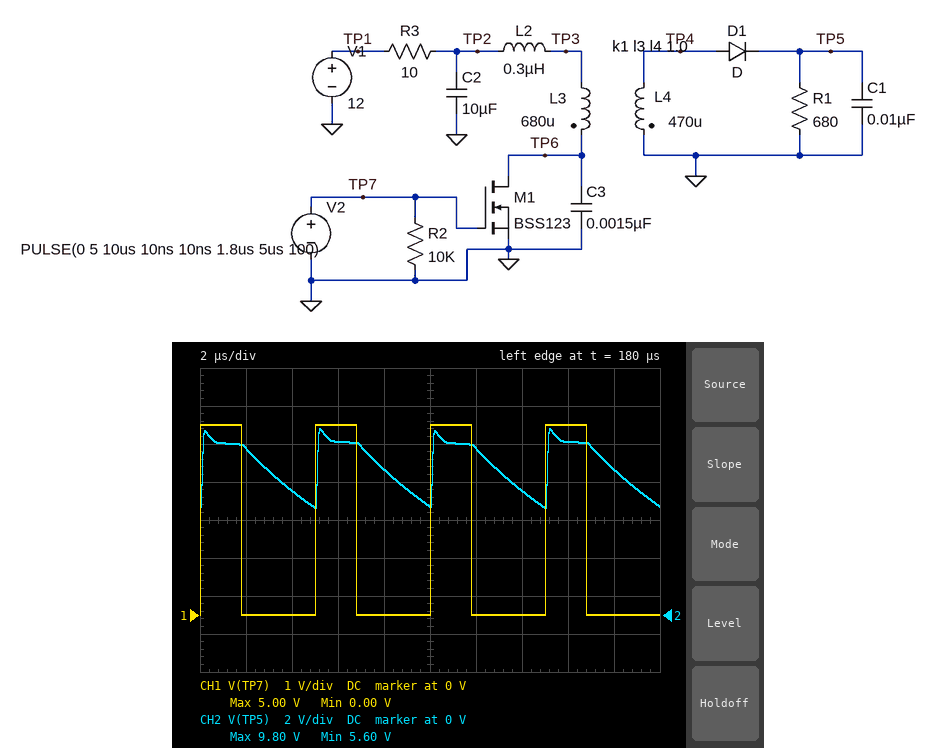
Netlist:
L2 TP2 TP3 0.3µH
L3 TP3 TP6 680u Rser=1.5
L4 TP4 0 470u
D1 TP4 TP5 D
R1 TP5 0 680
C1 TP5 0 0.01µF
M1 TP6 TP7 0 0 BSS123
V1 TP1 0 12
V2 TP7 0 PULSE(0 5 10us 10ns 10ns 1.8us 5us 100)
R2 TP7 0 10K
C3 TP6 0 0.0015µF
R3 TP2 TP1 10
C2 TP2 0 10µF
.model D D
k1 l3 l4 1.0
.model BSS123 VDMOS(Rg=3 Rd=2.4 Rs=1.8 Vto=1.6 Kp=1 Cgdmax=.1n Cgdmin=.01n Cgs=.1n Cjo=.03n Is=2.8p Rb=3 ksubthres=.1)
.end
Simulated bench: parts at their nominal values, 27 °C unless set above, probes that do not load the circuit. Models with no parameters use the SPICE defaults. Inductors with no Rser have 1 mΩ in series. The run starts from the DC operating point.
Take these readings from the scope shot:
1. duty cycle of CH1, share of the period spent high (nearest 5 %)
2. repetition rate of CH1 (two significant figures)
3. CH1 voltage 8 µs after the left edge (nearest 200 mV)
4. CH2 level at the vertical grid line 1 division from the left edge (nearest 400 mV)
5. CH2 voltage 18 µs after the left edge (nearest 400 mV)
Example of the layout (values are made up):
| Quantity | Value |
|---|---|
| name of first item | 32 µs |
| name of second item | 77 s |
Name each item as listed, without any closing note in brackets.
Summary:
| Quantity | Value |
|---|---|
| duty cycle of CH1, share of the period spent high | 35 % |
| repetition rate of CH1 | 200 kHz |
| CH1 voltage 8 µs after the left edge | 0 V |
| CH2 level at the vertical grid line 1 division from the left edge | 8.8 V |
| CH2 voltage 18 µs after the left edge | 7.6 V |
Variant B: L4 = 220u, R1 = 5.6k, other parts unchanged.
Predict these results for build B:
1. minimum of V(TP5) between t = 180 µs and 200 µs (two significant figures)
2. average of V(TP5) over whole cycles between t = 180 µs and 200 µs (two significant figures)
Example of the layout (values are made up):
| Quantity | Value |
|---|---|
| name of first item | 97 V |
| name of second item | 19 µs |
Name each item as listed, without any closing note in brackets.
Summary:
| Quantity | Value |
|---|---|
| minimum of V(TP5) between t = 180 µs and 200 µs | 5.7 V |
| average of V(TP5) over whole cycles between t = 180 µs and 200 µs | 6.0 V |
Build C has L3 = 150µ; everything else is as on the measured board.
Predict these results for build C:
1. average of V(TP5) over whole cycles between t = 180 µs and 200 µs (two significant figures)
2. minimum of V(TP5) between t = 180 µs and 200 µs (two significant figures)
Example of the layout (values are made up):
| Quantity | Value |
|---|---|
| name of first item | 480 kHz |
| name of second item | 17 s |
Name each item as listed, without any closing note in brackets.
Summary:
| Quantity | Value |
|---|---|
| average of V(TP5) over whole cycles between t = 180 µs and 200 µs | 17 V |
| minimum of V(TP5) between t = 180 µs and 200 µs | 14 V |
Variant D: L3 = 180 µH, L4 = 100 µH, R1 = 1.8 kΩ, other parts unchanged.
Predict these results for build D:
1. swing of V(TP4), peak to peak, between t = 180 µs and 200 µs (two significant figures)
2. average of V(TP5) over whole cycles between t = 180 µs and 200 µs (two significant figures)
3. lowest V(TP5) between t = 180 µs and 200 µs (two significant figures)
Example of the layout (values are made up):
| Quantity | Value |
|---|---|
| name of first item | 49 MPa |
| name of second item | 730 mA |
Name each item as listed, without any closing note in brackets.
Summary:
| Quantity | Value |
|---|---|
| swing of V(TP4), peak to peak, between t = 180 µs and 200 µs | 37 V |
| average of V(TP5) over whole cycles between t = 180 µs and 200 µs | 8.1 V |
| lowest V(TP5) between t = 180 µs and 200 µs | 7.1 V |
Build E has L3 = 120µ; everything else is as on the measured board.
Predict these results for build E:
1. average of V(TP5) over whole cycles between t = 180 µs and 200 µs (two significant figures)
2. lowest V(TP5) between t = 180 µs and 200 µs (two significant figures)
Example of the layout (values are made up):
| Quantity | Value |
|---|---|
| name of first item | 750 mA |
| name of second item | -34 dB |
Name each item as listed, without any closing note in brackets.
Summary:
| Quantity | Value |
|---|---|
| average of V(TP5) over whole cycles between t = 180 µs and 200 µs | 19 V |
| lowest V(TP5) between t = 180 µs and 200 µs | 16 V |
